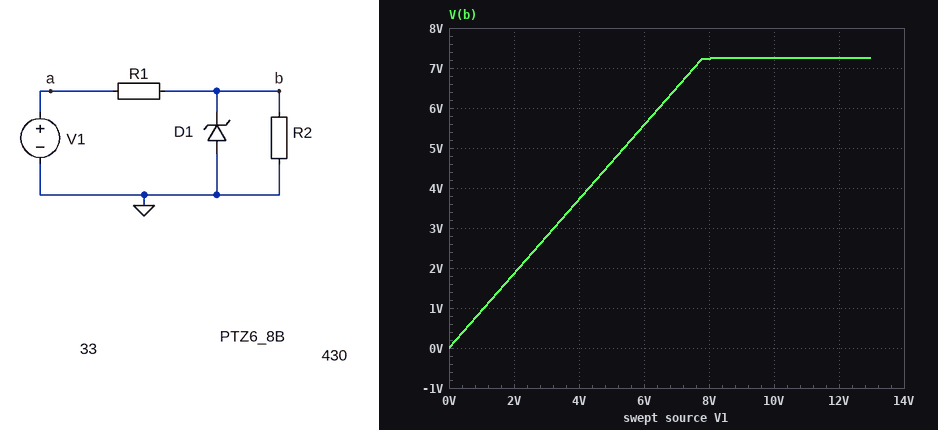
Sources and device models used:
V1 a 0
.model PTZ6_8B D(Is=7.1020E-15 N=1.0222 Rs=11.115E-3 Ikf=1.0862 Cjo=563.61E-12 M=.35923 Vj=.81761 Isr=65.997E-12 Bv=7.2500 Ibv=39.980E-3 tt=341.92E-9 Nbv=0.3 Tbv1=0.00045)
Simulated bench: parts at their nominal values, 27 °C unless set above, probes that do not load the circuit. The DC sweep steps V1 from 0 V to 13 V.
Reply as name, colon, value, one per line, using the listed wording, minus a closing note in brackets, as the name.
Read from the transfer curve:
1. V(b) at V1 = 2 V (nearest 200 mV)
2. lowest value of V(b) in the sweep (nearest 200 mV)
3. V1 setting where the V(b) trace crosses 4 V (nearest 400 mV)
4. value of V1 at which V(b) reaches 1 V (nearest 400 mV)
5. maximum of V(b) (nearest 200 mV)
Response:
V(b) at V1 = 2 V: 1.8 V
lowest value of V(b) in the sweep: 0 V
V1 setting where the V(b) trace crosses 4 V: 4.4 V
value of V1 at which V(b) reaches 1 V: 1.2 V
maximum of V(b): 7.2 V
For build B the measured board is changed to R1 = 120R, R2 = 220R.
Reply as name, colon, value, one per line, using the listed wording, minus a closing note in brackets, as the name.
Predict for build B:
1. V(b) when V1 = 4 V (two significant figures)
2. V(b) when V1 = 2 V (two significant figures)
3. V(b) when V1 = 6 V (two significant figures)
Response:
V(b) when V1 = 4 V: 2.6 V
V(b) when V1 = 2 V: 1.3 V
V(b) when V1 = 6 V: 3.9 V
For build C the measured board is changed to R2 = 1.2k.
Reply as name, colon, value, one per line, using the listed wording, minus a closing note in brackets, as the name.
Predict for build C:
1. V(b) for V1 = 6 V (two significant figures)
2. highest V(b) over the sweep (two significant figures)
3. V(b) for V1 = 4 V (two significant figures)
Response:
V(b) for V1 = 6 V: 5.8 V
highest V(b) over the sweep: 7.3 V
V(b) for V1 = 4 V: 3.9 V
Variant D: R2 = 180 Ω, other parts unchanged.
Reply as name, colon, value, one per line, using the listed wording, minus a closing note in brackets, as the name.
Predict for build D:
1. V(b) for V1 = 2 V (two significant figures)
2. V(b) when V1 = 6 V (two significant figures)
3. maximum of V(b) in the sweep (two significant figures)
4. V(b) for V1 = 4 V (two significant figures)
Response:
V(b) for V1 = 2 V: 1.7 V
V(b) when V1 = 6 V: 5.1 V
maximum of V(b) in the sweep: 7.3 V
V(b) for V1 = 4 V: 3.4 V
